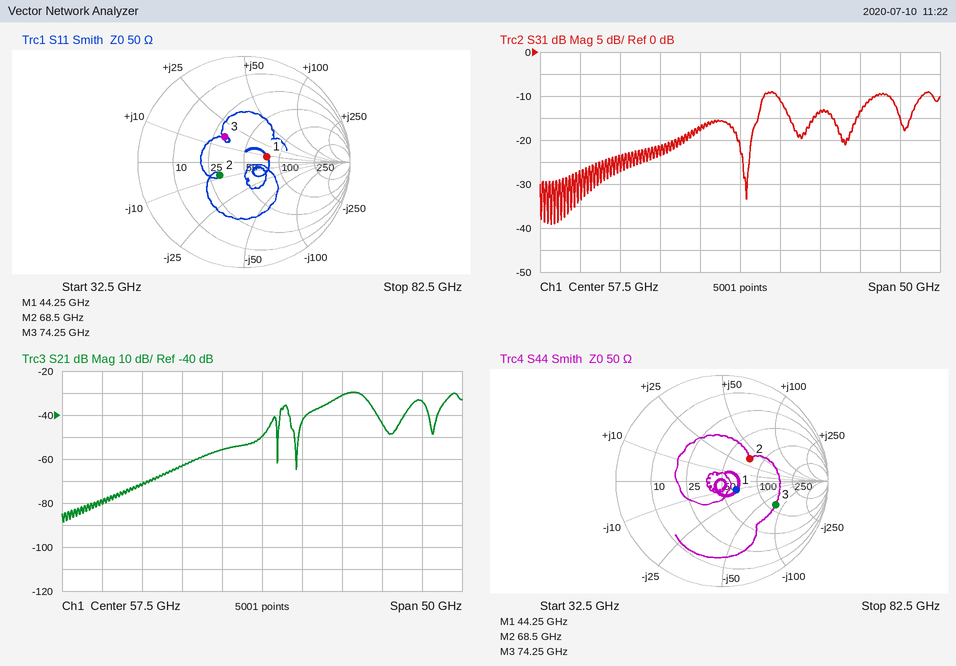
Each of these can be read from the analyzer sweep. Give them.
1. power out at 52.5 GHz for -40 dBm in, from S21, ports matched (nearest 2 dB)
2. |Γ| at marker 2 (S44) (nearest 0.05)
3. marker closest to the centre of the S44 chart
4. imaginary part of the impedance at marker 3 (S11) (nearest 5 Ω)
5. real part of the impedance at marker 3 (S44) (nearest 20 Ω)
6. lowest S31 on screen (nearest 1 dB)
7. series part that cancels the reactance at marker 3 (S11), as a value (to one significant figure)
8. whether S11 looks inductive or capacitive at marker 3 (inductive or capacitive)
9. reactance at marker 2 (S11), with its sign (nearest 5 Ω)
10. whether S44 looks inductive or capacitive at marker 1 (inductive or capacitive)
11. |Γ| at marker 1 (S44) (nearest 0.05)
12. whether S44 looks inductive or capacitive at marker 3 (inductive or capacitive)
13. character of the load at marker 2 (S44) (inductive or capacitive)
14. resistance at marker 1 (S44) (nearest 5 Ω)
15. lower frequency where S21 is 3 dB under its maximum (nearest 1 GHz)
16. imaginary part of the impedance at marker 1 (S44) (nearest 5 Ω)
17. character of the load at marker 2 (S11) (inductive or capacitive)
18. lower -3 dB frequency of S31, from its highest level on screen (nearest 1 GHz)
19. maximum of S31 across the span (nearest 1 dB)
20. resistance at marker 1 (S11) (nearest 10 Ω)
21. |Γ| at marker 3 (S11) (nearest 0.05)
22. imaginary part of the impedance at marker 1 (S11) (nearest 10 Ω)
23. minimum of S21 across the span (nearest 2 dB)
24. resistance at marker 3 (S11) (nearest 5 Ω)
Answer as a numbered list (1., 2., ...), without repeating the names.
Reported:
1. -96 dBm
2. 0.35
3. marker 1
4. +15 Ω
5. 120 Ω
6. -39 dB
7. 100 fF
8. inductive
9. -10 Ω
10. capacitive
11. 0.15
12. capacitive
13. inductive
14. 65 Ω
15. 67 GHz
16. -10 Ω
17. capacitive
18. 60 GHz
19. -9 dB
20. 80 Ω
21. 0.30
22. +10 Ω
23. -88 dB
24. 30 Ω
